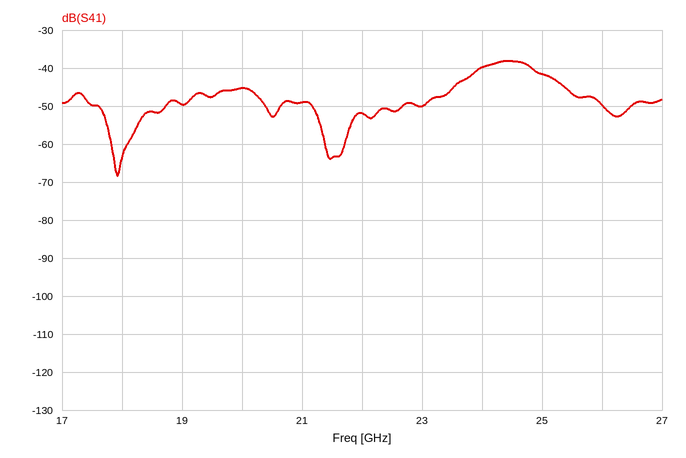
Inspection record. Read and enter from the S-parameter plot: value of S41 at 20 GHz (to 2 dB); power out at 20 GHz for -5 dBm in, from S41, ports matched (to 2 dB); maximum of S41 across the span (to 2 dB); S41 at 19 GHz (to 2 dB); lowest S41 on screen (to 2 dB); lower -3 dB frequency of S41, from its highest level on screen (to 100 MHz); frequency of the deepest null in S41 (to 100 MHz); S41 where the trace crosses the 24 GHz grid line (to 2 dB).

-46 dB
-50 dBm
-38 dB
-50 dB
-68 dB
23.9 GHz
17.9 GHz
-40 dB
